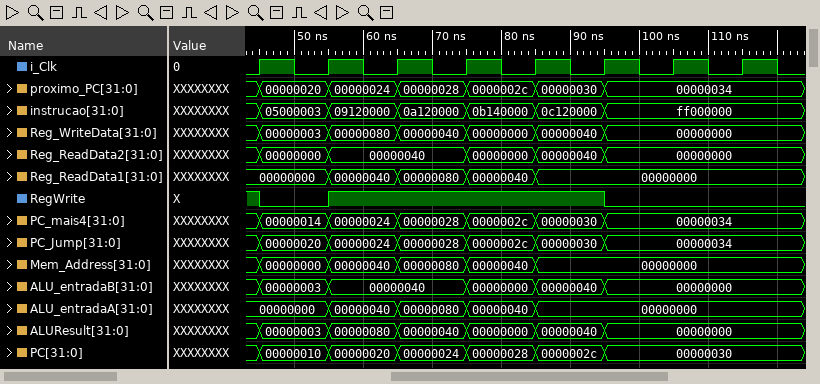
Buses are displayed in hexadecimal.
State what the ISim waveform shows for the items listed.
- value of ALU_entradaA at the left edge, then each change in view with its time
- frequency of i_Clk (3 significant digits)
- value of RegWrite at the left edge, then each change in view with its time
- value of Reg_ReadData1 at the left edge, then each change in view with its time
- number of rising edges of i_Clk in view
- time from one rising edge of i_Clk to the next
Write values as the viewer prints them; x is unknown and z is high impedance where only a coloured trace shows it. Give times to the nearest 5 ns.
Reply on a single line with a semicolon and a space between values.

00000000, 00000040 at 55 ns, 00000080 at 65 ns, 00000040 at 75 ns, 00000000 at 85 ns; 100 MHz; 1, 0 at 45 ns, 1 at 55 ns, 0 at 95 ns; 00000000, 00000040 at 55 ns, 00000080 at 65 ns, 00000040 at 75 ns, 00000000 at 85 ns; 8; 10 ns
